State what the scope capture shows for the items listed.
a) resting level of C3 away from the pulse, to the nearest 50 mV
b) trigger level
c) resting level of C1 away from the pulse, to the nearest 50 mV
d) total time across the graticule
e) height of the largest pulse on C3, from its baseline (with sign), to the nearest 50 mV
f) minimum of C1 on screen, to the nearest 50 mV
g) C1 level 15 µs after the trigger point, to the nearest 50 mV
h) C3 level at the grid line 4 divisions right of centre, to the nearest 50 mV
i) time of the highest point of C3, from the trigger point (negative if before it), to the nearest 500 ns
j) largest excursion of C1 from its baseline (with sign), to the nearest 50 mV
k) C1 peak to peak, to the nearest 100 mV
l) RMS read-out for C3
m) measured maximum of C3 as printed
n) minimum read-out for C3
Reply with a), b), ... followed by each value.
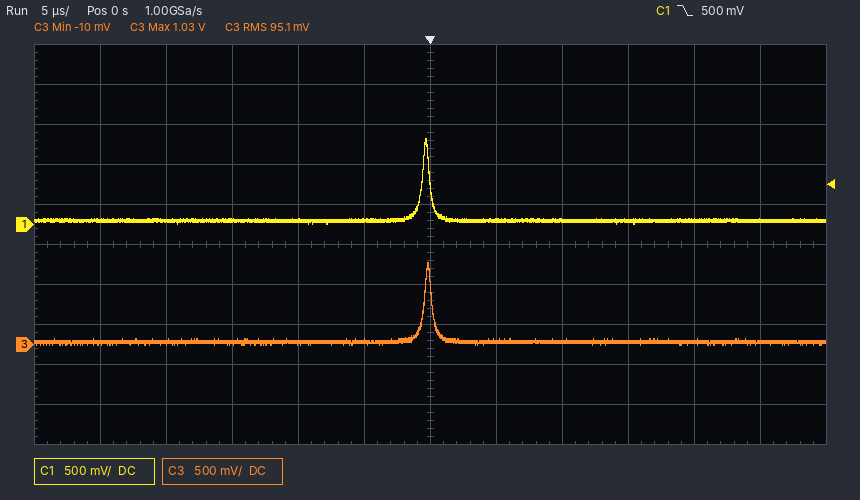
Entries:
a) 50 mV
b) 500 mV
c) 50 mV
d) 60 µs
e) +1.00 V
f) 0 mV
g) 50 mV
h) 50 mV
i) 0.0 µs
j) +1.05 V
k) 1.10 V
l) 95.1 mV
m) 1.03 V
n) -10 mV
